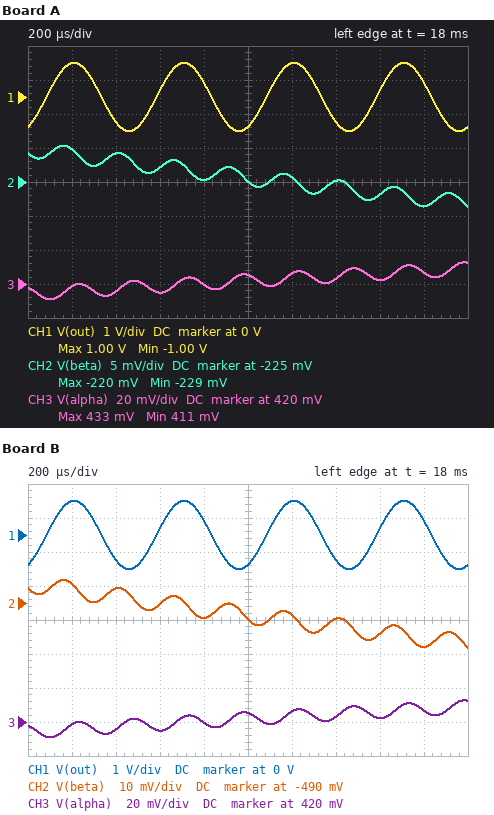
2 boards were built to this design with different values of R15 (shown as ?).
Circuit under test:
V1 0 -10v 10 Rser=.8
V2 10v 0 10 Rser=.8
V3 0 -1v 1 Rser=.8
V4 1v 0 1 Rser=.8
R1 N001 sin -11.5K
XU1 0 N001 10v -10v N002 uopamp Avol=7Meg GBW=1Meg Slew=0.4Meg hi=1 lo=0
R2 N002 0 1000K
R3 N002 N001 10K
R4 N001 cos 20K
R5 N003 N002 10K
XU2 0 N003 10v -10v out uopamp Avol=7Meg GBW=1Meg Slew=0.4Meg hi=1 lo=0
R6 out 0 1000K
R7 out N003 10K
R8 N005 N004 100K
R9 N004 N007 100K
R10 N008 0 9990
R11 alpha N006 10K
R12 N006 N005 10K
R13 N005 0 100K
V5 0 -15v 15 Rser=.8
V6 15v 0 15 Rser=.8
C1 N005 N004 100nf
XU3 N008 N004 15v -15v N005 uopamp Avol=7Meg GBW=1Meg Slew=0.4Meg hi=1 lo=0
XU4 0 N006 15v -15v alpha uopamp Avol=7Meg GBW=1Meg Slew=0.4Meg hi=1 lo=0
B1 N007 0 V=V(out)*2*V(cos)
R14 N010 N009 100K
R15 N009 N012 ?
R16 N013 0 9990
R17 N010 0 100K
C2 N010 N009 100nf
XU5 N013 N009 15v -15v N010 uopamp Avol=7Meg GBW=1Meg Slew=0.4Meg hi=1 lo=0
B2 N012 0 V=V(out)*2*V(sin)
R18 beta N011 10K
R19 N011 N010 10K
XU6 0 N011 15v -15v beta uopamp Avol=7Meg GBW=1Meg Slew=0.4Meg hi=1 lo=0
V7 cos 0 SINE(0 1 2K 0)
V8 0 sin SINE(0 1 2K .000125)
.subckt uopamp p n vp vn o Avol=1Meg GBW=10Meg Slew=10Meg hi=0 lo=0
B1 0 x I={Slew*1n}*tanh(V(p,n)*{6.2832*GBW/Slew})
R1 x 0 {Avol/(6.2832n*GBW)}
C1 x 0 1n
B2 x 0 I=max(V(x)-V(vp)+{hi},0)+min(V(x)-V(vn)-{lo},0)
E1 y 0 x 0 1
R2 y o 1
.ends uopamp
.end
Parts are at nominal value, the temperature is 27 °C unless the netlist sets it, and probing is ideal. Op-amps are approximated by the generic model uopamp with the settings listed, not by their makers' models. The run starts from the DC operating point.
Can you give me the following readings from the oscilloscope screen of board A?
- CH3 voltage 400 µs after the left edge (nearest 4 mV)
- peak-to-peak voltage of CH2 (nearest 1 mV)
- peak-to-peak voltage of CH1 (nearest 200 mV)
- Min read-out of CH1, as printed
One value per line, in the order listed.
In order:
416 mV
9 mV
2.0 V
-1.00 V
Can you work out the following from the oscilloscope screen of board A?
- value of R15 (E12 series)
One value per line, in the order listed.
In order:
330 kΩ
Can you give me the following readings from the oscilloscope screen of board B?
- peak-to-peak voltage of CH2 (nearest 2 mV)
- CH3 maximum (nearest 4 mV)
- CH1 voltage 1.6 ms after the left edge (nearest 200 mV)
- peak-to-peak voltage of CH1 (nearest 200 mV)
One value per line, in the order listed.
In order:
20 mV
432 mV
200 mV
2.0 V
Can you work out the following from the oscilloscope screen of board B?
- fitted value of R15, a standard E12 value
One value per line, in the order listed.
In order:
150 kΩ
